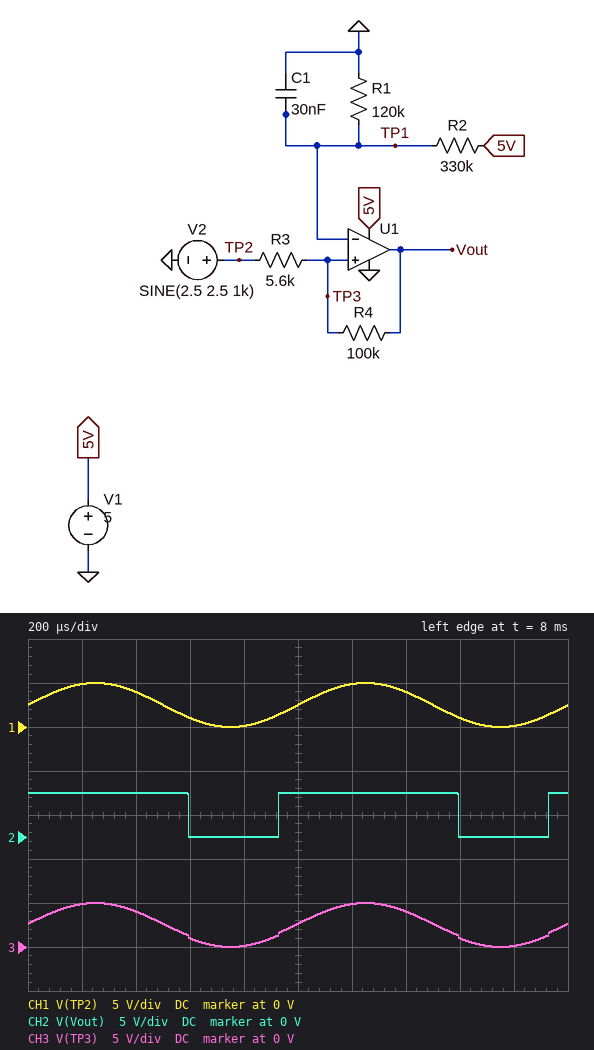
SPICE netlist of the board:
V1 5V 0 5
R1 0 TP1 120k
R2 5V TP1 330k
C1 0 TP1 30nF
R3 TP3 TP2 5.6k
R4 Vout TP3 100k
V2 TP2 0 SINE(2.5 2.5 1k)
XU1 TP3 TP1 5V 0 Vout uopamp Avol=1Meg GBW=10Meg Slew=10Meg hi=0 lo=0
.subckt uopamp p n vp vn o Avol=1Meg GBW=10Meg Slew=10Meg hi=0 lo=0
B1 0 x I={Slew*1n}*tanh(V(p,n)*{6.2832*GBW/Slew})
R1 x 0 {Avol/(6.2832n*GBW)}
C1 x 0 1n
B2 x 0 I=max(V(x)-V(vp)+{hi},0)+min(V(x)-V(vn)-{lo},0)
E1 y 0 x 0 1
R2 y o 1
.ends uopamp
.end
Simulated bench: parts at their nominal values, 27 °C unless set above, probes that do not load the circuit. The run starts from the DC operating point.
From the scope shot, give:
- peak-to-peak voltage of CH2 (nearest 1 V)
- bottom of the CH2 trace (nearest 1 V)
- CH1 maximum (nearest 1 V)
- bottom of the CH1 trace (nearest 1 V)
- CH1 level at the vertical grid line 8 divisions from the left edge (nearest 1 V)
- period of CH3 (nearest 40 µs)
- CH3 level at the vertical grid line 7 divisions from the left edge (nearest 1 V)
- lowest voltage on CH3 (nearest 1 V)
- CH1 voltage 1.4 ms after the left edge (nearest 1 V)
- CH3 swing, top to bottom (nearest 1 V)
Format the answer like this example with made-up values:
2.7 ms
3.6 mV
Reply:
5 V
0 V
5 V
0 V
1 V
1.00 ms
4 V
0 V
4 V
5 V
